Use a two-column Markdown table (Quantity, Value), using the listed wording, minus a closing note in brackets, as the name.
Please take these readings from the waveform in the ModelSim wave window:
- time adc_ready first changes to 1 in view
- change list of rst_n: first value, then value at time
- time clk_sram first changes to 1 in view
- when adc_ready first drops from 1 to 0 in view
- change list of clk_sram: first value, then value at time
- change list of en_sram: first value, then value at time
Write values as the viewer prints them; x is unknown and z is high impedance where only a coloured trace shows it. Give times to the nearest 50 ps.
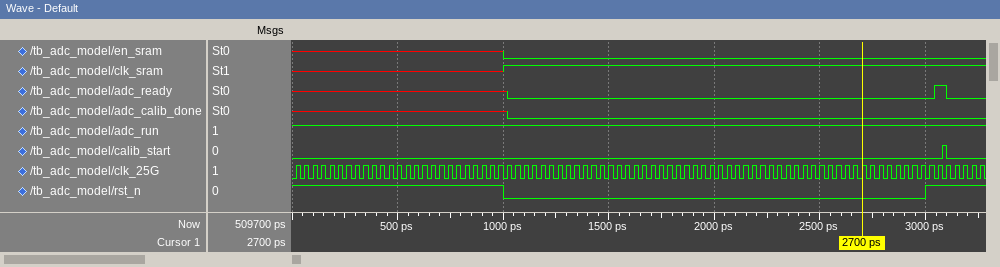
| Quantity | Value |
|---|---|
| time adc_ready first changes to 1 in view | 3050 ps |
| change list of rst_n: first value, then value at time | 1, 0 at 1000 ps, 1 at 3000 ps |
| time clk_sram first changes to 1 in view | 1000 ps |
| when adc_ready first drops from 1 to 0 in view | 3100 ps |
| change list of clk_sram: first value, then value at time | x, 1 at 1000 ps |
| change list of en_sram: first value, then value at time | x, 0 at 1000 ps |
